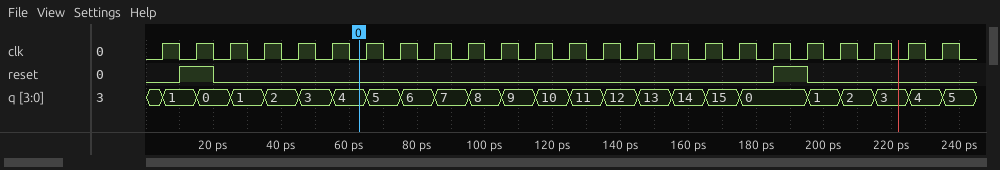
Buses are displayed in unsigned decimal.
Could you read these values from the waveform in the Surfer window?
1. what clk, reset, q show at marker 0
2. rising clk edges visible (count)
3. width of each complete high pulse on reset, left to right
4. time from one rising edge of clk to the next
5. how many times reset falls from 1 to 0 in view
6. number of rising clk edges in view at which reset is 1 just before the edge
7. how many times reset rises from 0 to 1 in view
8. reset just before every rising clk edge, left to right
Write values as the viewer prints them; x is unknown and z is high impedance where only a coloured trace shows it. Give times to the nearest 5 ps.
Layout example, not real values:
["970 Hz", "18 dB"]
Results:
["clk=0, reset=0, q=4", "24", "10 ps, 10 ps", "10 ps", "2", "2", "2", "0 1 0 0 0 0 0 0 0 0 0 0 0 0 0 0 0 0 0 1 0 0 0 0"]
